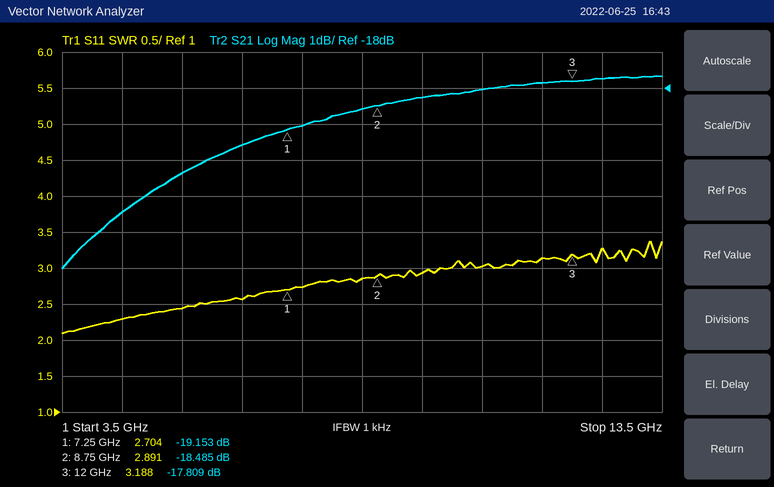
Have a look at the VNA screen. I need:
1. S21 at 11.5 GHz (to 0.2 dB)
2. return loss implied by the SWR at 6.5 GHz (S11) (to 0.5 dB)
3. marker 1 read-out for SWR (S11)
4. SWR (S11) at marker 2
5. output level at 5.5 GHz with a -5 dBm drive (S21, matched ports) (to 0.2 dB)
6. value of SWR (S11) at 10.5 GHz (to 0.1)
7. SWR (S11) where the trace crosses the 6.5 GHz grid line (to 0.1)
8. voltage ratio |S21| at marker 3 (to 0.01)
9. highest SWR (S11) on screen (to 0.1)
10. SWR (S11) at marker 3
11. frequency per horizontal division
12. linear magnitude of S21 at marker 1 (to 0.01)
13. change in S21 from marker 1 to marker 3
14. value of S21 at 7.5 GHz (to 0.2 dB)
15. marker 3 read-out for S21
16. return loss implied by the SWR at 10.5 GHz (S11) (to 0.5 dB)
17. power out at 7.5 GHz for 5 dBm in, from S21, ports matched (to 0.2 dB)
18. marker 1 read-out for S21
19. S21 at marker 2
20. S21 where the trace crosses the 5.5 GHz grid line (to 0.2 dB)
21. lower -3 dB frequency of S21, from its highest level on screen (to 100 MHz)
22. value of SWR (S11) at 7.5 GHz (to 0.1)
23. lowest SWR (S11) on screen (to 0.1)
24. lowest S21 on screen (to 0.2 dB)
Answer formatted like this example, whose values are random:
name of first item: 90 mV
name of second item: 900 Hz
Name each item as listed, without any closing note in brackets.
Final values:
S21 at 11.5 GHz: -17.8 dB
return loss implied by the SWR at 6.5 GHz (S11): 7.0 dB
marker 1 read-out for SWR: 2.704
SWR (S11) at marker 2: 2.891
output level at 5.5 GHz with a -5 dBm drive (S21, matched ports): -25.4 dBm
value of SWR (S11) at 10.5 GHz: 3.0
SWR (S11) where the trace crosses the 6.5 GHz grid line: 2.6
voltage ratio |S21| at marker 3: 0.13
highest SWR (S11) on screen: 3.4
SWR (S11) at marker 3: 3.188
frequency per horizontal division: 1 GHz
linear magnitude of S21 at marker 1: 0.11
change in S21 from marker 1 to marker 3: 1.344 dB
value of S21 at 7.5 GHz: -19.0 dB
marker 3 read-out for S21: -17.809 dB
return loss implied by the SWR at 10.5 GHz (S11): 6.0 dB
power out at 7.5 GHz for 5 dBm in, from S21, ports matched: -14.0 dBm
marker 1 read-out for S21: -19.153 dB
S21 at marker 2: -18.485 dB
S21 where the trace crosses the 5.5 GHz grid line: -20.4 dB
lower -3 dB frequency of S21, from its highest level on screen: 5.2 GHz
value of SWR (S11) at 7.5 GHz: 2.7
lowest SWR (S11) on screen: 2.1
lowest S21 on screen: -23.0 dB
